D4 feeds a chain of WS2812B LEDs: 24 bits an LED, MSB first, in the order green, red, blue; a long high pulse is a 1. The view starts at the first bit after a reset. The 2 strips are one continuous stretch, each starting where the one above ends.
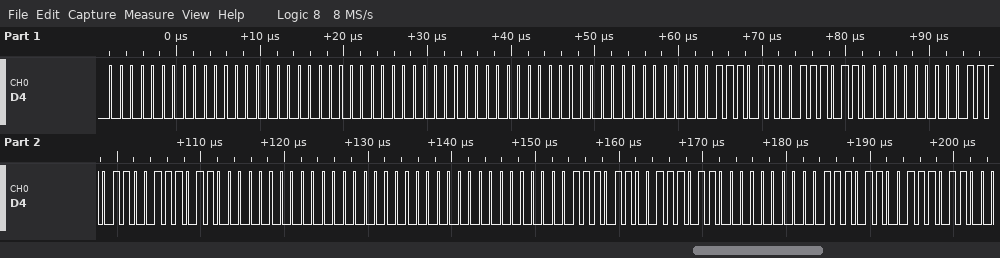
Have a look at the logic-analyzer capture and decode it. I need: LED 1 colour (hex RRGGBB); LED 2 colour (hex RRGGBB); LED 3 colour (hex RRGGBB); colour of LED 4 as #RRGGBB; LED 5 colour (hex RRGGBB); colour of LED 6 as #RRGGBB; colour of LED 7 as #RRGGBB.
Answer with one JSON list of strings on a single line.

["#000000", "#000000", "#3B003B", "#3B003B", "#000000", "#3B003B", "#3B003B"]
